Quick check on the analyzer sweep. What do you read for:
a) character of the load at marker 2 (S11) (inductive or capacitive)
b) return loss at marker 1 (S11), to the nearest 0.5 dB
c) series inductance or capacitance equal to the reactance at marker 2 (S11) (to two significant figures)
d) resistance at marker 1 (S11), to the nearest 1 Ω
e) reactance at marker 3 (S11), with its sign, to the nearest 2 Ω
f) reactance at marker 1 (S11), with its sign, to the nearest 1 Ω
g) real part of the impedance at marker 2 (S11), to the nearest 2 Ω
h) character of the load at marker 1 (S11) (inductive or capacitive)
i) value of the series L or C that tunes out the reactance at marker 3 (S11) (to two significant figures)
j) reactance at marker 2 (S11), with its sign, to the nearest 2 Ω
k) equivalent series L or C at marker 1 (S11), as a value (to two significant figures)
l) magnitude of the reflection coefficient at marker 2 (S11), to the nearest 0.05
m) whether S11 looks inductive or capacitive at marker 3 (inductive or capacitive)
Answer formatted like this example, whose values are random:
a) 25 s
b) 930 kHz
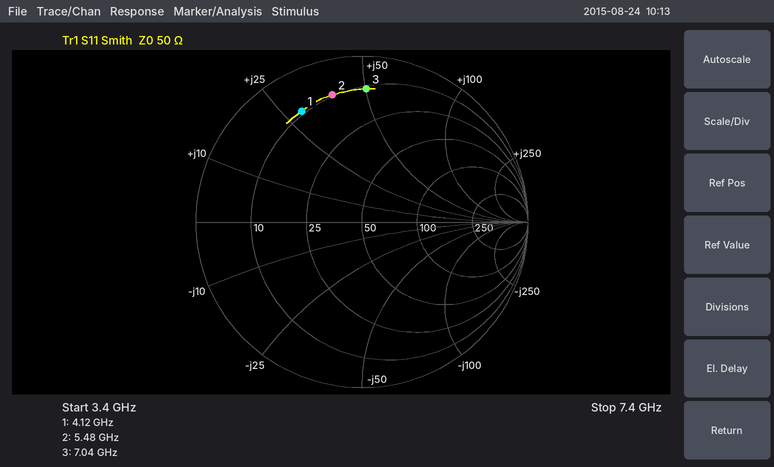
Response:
a) inductive
b) 2.5 dB
c) 1.1 nH
d) 9 Ω
e) +50 Ω
f) +29 Ω
g) 10 Ω
h) inductive
i) 450 fF
j) +38 Ω
k) 1.1 nH
l) 0.80
m) inductive
